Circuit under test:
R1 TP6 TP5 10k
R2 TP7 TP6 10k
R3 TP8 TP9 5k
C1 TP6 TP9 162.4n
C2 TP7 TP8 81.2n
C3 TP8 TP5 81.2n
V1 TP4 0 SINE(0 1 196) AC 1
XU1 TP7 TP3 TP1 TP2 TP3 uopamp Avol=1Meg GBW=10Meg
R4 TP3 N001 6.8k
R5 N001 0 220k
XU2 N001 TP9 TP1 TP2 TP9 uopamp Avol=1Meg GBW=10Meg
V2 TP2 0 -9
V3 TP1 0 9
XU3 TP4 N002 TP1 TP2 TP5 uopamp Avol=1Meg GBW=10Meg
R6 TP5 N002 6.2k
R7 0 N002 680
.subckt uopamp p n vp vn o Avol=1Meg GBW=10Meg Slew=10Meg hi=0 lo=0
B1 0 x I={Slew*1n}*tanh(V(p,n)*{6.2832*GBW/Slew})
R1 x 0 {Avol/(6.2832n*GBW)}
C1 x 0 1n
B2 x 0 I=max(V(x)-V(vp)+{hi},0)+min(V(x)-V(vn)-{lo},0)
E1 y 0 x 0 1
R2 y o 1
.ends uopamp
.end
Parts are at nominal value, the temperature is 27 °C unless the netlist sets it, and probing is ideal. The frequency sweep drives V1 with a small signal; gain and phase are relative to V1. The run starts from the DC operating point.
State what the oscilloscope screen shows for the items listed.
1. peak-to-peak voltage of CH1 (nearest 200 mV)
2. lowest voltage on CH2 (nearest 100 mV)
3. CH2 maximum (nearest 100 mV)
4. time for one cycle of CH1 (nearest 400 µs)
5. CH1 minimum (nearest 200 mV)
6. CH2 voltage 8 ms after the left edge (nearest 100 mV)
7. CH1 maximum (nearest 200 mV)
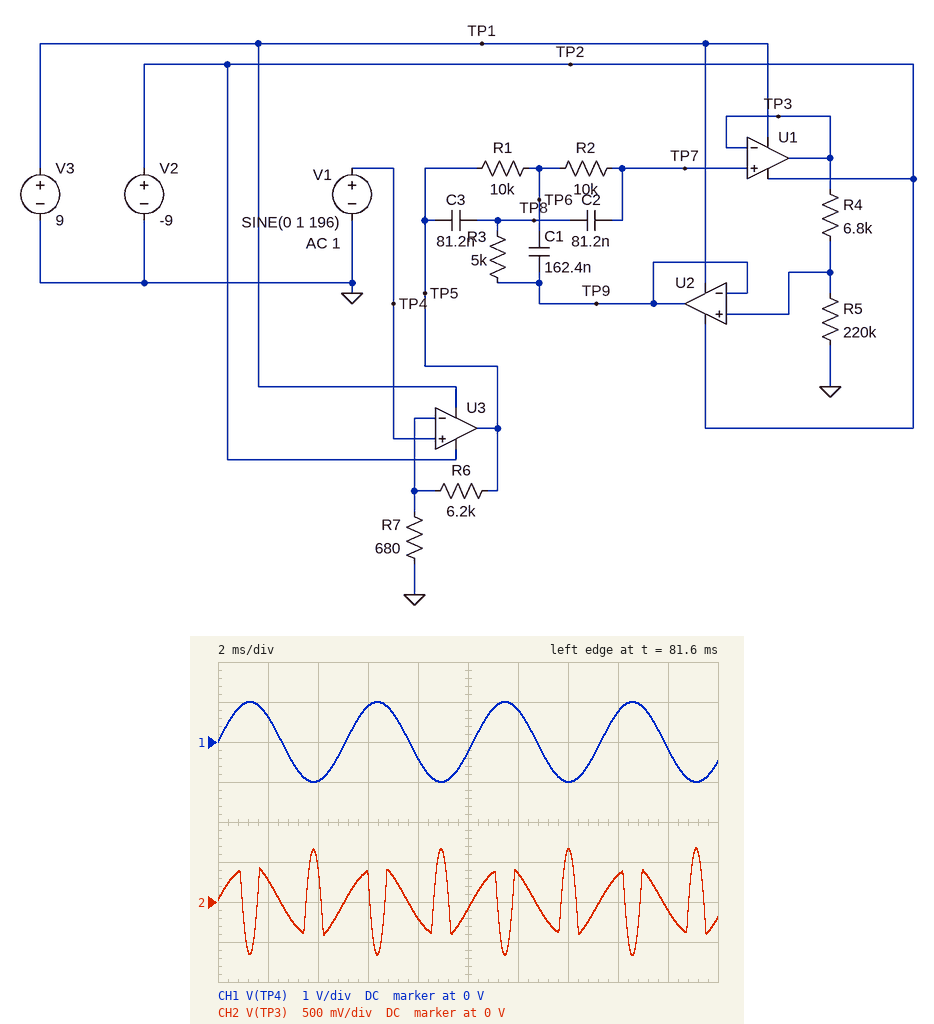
2.0 V
-700 mV
700 mV
5.2 ms
-1.0 V
-200 mV
1.0 V
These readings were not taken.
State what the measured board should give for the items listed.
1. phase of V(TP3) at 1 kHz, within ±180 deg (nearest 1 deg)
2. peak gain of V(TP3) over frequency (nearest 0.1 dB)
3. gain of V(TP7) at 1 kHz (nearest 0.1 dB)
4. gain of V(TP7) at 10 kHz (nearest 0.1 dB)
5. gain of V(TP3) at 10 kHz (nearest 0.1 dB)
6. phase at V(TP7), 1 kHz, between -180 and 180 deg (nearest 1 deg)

1 deg
20.1 dB
20.1 dB
20.1 dB
20.1 dB
1 deg
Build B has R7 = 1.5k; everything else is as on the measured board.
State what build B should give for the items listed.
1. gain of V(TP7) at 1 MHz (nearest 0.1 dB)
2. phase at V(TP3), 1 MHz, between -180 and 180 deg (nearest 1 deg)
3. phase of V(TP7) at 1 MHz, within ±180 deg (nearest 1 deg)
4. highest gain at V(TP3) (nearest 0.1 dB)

13.2 dB
-33 deg
-27 deg
14.2 dB
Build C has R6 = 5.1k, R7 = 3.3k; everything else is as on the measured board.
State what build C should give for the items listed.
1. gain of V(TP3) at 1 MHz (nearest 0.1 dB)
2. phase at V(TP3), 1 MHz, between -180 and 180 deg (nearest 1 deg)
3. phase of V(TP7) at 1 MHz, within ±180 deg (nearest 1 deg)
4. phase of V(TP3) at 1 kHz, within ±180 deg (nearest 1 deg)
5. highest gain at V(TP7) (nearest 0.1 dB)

7.8 dB
-20 deg
-14 deg
1 deg
8.1 dB
